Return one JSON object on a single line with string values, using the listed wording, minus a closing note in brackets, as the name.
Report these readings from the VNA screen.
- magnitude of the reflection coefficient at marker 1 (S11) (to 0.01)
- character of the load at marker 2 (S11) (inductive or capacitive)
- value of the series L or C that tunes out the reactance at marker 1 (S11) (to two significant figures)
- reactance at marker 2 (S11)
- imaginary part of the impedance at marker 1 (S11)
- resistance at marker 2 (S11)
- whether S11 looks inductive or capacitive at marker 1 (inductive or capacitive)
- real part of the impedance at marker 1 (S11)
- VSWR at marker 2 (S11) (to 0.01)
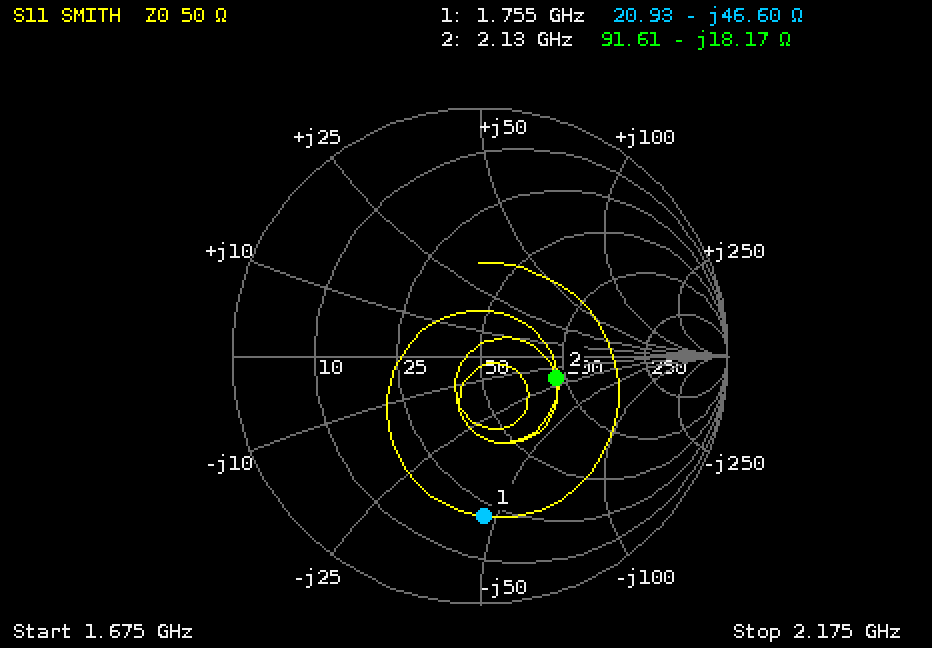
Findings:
{"magnitude of the reflection coefficient at marker 1 (S11)": "0.65", "character of the load at marker 2 (S11)": "capacitive", "value of the series L or C that tunes out the reactance at marker 1 (S11)": "4.2 nH", "reactance at marker 2": "-18.17 Ω", "imaginary part of the impedance at marker 1": "-46.60 Ω", "resistance at marker 2": "91.61 Ω", "whether S11 looks inductive or capacitive at marker 1": "capacitive", "real part of the impedance at marker 1": "20.93 Ω", "VSWR at marker 2 (S11)": "1.93"}
